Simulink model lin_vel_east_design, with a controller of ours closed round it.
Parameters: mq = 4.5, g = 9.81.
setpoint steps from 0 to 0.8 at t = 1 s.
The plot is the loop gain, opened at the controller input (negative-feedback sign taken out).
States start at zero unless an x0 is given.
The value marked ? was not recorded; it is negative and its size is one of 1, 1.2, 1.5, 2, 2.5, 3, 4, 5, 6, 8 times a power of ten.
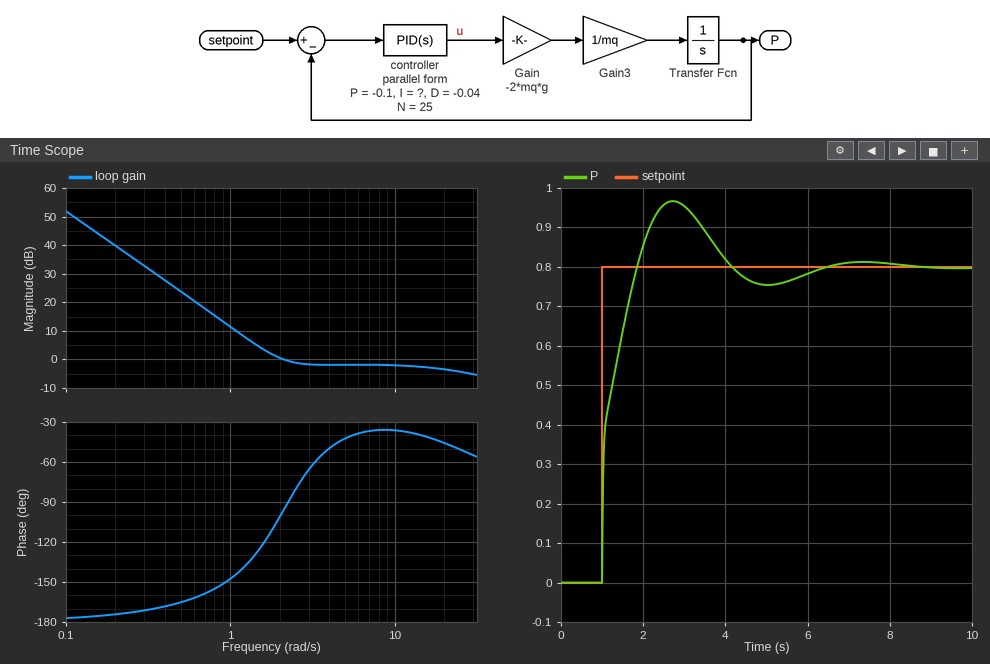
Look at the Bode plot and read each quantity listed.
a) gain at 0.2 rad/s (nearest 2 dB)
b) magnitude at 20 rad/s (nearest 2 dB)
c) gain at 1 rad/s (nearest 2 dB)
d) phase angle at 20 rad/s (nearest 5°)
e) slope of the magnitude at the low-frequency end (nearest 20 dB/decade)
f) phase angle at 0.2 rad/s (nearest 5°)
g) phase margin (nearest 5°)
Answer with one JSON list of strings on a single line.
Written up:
["40 dB", "-4 dB", "12 dB", "-45°", "-40 dB/decade", "-175°", "85°"]
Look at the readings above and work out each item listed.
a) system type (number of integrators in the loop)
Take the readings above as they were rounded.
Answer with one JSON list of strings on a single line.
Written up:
["2"]
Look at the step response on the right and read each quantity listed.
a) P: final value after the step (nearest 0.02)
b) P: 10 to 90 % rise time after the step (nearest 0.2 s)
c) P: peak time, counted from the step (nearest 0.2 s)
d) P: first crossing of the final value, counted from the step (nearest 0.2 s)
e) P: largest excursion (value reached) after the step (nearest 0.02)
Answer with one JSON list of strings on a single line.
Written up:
["0.80", "0.6 s", "1.8 s", "0.8 s", "0.96"]
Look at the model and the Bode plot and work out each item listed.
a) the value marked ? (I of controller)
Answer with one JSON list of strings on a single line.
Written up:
["-0.2"]
